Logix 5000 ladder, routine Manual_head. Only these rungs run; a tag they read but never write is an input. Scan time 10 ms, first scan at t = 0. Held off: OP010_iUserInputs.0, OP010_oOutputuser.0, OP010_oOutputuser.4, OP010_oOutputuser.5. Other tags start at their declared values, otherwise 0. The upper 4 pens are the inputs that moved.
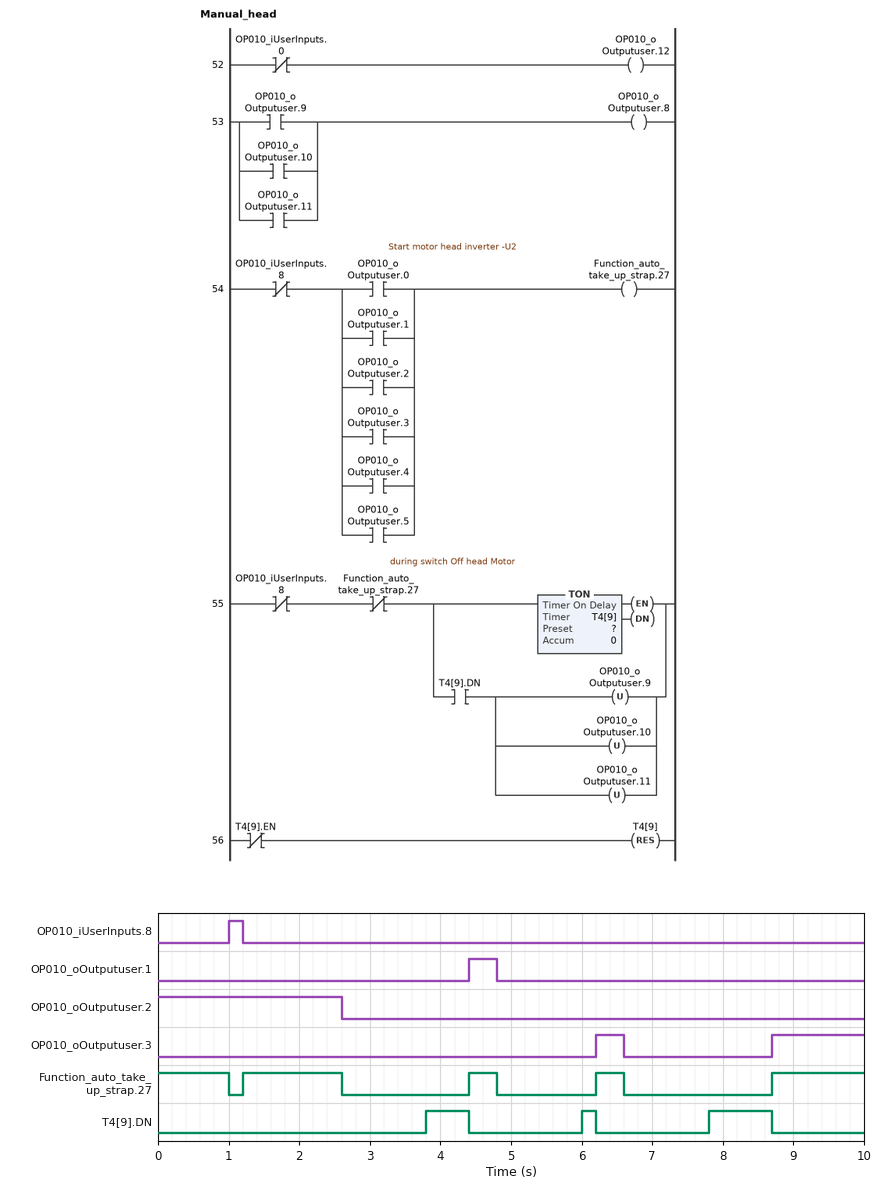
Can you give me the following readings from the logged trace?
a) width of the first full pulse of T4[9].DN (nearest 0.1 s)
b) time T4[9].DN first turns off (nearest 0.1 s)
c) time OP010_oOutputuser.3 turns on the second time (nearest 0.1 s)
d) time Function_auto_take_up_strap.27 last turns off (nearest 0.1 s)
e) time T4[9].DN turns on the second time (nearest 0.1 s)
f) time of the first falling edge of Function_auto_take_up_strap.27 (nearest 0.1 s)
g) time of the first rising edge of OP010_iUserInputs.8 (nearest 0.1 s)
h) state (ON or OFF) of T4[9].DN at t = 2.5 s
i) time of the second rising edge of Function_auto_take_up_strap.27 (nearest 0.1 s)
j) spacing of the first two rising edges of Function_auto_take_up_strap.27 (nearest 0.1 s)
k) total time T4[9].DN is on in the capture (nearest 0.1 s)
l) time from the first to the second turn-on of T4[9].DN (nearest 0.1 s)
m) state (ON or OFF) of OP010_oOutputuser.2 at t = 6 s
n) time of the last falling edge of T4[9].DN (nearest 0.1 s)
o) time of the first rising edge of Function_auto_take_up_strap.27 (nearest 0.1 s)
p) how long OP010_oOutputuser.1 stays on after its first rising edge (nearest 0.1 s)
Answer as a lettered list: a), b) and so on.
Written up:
a) 0.6 s
b) 4.4 s
c) 8.7 s
d) 6.6 s
e) 6.0 s
f) 1.0 s
g) 1.0 s
h) OFF
i) 4.4 s
j) 3.2 s
k) 1.7 s
l) 2.2 s
m) OFF
n) 8.7 s
o) 1.2 s
p) 0.4 s
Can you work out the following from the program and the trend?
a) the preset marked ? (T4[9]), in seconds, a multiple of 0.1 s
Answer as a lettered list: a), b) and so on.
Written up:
a) 1.2 s
